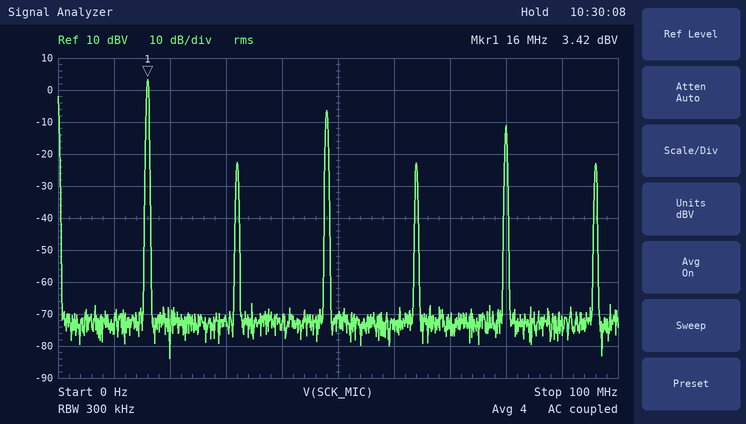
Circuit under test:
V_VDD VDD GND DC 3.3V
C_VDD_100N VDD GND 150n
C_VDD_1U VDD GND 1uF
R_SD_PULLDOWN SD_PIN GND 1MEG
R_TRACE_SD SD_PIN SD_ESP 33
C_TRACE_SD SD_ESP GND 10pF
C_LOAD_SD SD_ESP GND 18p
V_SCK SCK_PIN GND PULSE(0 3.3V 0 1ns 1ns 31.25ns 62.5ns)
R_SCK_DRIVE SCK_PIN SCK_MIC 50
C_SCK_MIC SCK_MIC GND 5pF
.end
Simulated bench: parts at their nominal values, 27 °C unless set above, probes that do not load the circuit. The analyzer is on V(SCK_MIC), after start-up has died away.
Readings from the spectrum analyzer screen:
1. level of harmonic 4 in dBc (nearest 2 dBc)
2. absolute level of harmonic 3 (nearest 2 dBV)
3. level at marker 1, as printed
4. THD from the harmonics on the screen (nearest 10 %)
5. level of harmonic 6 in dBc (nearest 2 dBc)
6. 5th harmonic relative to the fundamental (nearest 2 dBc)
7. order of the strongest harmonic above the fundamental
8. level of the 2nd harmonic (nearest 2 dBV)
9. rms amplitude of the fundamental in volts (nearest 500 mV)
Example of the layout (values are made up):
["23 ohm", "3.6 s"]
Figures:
["-26 dBc", "-6 dBV", "3.42 dBV", "40 %", "-26 dBc", "-14 dBc", "3", "-22 dBV", "1.5 V"]
